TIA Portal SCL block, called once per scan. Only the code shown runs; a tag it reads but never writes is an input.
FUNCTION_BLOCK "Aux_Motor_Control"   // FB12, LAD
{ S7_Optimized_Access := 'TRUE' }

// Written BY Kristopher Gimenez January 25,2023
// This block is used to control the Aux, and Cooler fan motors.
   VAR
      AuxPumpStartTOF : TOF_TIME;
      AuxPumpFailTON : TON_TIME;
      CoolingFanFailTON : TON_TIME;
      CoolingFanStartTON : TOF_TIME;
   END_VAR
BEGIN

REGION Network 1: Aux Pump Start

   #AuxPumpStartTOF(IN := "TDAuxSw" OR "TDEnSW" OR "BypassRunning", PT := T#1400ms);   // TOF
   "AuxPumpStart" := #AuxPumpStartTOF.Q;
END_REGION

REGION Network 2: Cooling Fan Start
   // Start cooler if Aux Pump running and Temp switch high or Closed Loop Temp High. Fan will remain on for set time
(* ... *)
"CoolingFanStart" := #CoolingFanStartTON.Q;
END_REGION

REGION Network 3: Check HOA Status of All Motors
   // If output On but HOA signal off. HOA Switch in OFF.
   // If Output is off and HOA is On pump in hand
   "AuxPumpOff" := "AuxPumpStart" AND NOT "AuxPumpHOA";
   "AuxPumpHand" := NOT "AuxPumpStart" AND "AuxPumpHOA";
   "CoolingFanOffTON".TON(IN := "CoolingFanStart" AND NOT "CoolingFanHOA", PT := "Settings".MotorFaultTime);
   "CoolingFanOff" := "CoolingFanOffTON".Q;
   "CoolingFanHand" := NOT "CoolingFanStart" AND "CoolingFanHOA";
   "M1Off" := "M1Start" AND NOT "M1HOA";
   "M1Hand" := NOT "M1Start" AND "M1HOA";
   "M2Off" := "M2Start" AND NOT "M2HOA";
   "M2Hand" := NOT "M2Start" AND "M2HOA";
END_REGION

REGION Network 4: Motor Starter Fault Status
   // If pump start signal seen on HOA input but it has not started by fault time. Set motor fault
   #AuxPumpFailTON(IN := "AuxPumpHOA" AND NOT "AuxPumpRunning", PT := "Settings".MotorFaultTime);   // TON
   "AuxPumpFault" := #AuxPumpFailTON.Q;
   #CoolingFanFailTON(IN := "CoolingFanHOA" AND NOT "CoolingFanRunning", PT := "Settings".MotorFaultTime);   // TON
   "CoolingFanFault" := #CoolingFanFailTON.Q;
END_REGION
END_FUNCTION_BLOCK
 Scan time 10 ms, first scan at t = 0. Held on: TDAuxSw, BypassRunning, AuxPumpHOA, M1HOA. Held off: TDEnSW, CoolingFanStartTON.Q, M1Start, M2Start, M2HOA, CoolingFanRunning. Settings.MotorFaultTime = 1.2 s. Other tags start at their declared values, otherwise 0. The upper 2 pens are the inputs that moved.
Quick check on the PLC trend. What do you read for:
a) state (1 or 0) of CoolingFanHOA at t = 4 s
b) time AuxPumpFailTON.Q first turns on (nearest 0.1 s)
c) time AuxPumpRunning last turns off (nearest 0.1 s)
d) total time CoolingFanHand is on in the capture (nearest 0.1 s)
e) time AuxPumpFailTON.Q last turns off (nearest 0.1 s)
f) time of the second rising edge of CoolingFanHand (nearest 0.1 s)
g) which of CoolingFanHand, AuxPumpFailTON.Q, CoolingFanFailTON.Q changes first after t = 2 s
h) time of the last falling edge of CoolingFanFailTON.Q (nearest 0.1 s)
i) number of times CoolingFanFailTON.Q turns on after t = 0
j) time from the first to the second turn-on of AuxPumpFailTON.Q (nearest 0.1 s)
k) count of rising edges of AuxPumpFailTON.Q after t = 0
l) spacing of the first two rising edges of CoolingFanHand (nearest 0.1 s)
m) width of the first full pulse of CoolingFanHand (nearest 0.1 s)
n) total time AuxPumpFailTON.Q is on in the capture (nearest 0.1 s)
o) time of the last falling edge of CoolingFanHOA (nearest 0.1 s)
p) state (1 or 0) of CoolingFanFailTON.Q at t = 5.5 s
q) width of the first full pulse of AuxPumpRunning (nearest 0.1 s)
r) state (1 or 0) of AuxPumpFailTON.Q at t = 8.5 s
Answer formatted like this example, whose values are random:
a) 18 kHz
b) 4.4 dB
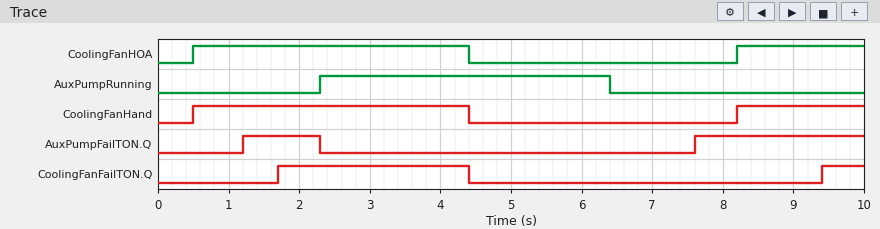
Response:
a) 1
b) 1.2 s
c) 6.4 s
d) 5.7 s
e) 2.3 s
f) 8.2 s
g) AuxPumpFailTON.Q
h) 4.4 s
i) 2
j) 6.4 s
k) 2
l) 7.7 s
m) 3.9 s
n) 3.5 s
o) 4.4 s
p) 0
q) 4.1 s
r) 1
